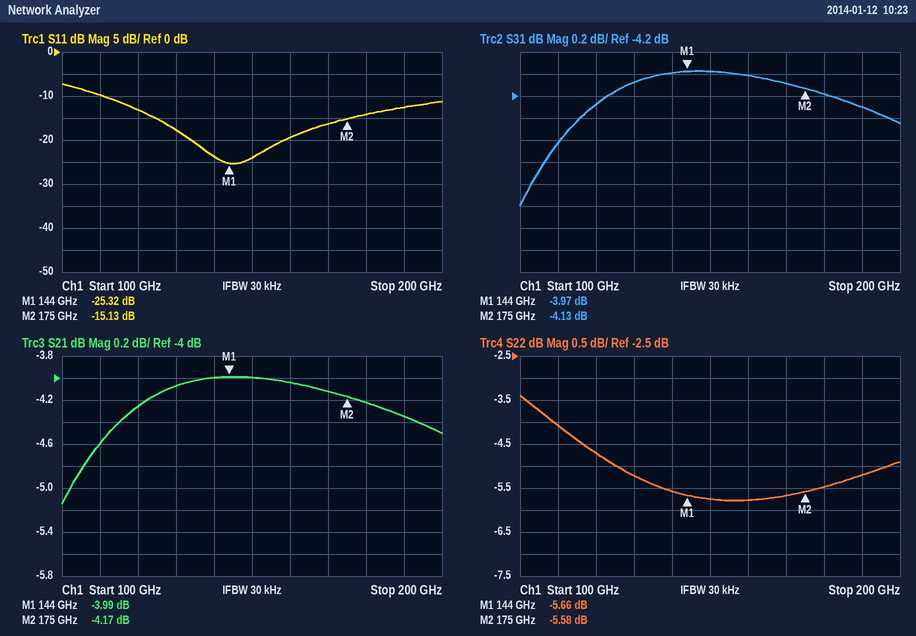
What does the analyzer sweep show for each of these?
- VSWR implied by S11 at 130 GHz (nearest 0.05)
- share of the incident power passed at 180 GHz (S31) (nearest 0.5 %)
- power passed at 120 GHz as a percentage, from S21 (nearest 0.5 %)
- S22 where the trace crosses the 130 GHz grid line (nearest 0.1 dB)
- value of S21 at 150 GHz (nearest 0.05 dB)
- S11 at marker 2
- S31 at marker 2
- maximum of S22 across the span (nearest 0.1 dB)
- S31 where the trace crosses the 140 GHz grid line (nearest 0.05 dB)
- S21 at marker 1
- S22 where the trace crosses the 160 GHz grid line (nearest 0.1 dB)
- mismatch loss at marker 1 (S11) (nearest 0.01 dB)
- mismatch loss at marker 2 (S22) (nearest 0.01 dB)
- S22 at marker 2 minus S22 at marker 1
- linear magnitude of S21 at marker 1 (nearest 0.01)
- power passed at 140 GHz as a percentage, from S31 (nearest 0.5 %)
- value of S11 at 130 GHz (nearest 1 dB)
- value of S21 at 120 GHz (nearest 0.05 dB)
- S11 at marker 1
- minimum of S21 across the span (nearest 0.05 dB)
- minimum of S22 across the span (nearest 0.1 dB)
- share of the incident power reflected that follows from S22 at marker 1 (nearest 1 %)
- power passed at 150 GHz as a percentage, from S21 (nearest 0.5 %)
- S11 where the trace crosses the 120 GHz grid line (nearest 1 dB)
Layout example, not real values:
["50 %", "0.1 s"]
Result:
["1.30", "38.0 %", "37.5 %", "-5.2 dB", "-4.00 dB", "-15.13 dB", "-4.13 dB", "-3.4 dB", "-4.00 dB", "-3.99 dB", "-5.8 dB", "0.01 dB", "1.41 dB", "0.08 dB", "0.63", "40.0 %", "-18 dB", "-4.25 dB", "-25.32 dB", "-5.15 dB", "-5.8 dB", "27 %", "40.0 %", "-13 dB"]
